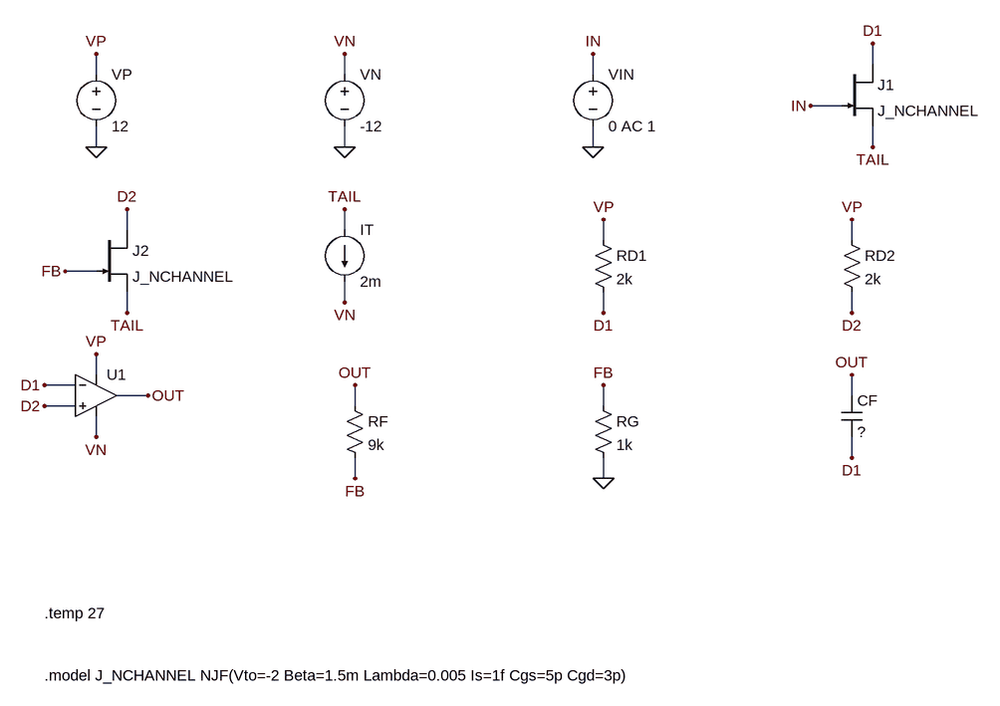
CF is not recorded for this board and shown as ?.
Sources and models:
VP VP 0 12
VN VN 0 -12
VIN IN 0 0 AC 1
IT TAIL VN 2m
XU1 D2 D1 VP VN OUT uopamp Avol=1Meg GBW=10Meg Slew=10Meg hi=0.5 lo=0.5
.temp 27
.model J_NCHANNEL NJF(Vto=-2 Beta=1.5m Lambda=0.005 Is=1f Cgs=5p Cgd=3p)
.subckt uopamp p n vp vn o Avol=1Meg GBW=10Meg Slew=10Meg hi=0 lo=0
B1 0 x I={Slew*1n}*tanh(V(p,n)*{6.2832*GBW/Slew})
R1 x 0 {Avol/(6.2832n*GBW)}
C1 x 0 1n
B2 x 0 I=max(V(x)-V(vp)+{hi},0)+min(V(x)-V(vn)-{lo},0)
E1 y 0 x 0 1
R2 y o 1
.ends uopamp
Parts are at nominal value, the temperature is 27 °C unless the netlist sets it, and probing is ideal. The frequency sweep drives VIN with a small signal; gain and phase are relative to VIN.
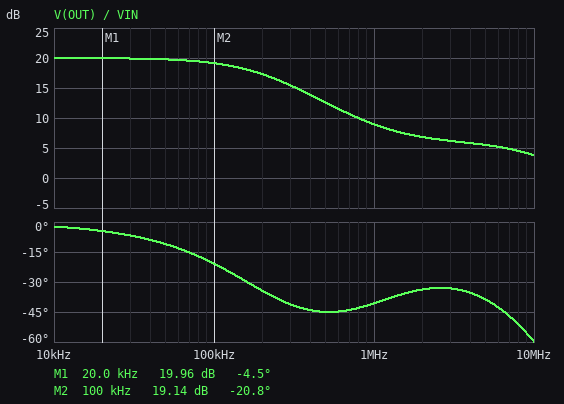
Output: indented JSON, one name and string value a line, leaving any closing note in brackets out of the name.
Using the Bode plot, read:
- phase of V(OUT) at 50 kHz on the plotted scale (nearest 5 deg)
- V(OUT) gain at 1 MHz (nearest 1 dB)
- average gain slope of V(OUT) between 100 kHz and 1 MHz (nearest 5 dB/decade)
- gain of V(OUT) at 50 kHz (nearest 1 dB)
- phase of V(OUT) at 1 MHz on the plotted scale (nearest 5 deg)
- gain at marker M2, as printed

{
  "phase of V(OUT) at 50 kHz on the plotted scale": "-10 deg",
  "V(OUT) gain at 1 MHz": "9 dB",
  "average gain slope of V(OUT) between 100 kHz and 1 MHz": "-10 dB/decade",
  "gain of V(OUT) at 50 kHz": "20 dB",
  "phase of V(OUT) at 1 MHz on the plotted scale": "-40 deg",
  "gain at marker M2, as printed": "19.14 dB"
}
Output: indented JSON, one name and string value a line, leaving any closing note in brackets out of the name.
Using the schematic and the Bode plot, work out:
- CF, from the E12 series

{
  "CF, from the E12 series": "150 pF"
}
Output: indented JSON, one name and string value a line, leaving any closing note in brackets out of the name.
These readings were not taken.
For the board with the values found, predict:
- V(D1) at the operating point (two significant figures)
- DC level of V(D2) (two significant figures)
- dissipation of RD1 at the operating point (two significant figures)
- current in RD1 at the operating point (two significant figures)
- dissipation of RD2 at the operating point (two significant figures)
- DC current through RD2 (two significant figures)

{
  "V(D1) at the operating point": "10 V",
  "DC level of V(D2)": "10 V",
  "dissipation of RD1 at the operating point": "2.0 mW",
  "current in RD1 at the operating point": "1.0 mA",
  "dissipation of RD2 at the operating point": "2.0 mW",
  "DC current through RD2": "1.0 mA"
}
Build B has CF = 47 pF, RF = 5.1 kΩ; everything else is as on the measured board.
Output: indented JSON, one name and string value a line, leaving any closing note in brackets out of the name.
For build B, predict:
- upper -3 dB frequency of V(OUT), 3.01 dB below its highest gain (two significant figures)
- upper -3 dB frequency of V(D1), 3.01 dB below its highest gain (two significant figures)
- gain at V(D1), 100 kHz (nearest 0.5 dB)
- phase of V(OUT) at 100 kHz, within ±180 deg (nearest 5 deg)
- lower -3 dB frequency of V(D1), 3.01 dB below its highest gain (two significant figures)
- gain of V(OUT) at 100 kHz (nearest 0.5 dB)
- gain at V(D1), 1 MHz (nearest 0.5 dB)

{
  "upper -3 dB frequency of V(OUT), 3.01 dB below its highest gain": "1.0 MHz",
  "upper -3 dB frequency of V(D1), 3.01 dB below its highest gain": "15 MHz",
  "gain at V(D1), 100 kHz": "-16.5 dB",
  "phase of V(OUT) at 100 kHz, within ±180 deg": "-5 deg",
  "lower -3 dB frequency of V(D1), 3.01 dB below its highest gain": "850 kHz",
  "gain of V(OUT) at 100 kHz": "15.5 dB",
  "gain at V(D1), 1 MHz": "0.5 dB"
}
